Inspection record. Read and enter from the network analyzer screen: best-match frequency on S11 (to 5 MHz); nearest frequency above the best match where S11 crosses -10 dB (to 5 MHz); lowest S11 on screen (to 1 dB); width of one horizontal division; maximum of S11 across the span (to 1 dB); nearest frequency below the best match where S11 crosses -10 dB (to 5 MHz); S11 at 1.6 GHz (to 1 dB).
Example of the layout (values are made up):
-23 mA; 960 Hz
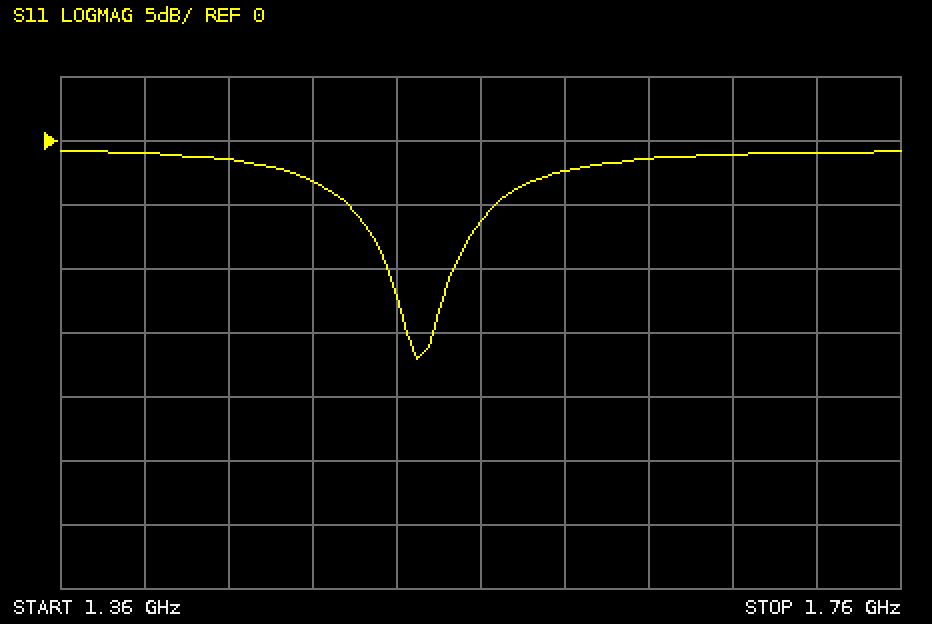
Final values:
1.530 GHz; 1.545 GHz; -17 dB; 40 MHz; -1 dB; 1.515 GHz; -2 dB
